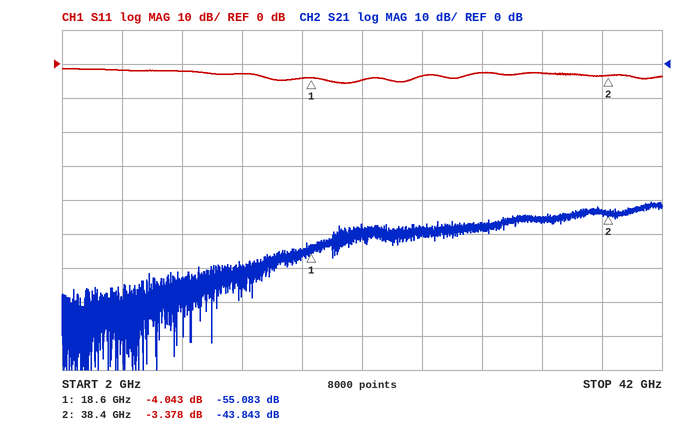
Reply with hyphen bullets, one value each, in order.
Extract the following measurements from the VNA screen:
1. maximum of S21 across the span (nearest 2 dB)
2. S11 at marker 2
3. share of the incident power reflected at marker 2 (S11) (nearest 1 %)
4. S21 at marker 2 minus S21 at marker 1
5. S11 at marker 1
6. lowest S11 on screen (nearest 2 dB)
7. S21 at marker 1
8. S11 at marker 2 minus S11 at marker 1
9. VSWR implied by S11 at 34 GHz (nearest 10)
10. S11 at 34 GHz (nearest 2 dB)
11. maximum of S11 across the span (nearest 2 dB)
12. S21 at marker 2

- -40 dB
- -3.378 dB
- 46 %
- 11.240 dB
- -4.043 dB
- -6 dB
- -55.083 dB
- 0.665 dB
- 10
- -2 dB
- -2 dB
- -43.843 dB
